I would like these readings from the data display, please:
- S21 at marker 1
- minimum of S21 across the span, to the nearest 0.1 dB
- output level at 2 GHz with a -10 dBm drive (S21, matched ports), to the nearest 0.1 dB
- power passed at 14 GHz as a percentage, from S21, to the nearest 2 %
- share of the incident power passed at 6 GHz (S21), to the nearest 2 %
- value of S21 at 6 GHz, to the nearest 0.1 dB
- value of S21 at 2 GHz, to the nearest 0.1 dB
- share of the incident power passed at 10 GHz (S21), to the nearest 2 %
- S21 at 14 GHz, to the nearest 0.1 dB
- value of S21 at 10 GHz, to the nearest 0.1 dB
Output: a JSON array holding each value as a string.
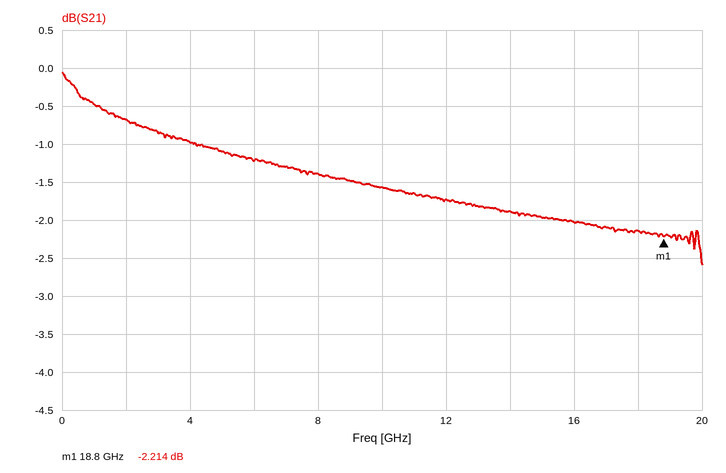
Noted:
["-2.214 dB", "-2.6 dB", "-10.7 dBm", "64 %", "76 %", "-1.2 dB", "-0.7 dB", "70 %", "-1.9 dB", "-1.6 dB"]
